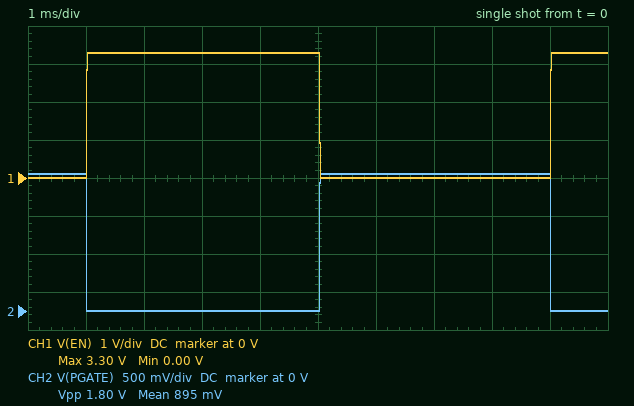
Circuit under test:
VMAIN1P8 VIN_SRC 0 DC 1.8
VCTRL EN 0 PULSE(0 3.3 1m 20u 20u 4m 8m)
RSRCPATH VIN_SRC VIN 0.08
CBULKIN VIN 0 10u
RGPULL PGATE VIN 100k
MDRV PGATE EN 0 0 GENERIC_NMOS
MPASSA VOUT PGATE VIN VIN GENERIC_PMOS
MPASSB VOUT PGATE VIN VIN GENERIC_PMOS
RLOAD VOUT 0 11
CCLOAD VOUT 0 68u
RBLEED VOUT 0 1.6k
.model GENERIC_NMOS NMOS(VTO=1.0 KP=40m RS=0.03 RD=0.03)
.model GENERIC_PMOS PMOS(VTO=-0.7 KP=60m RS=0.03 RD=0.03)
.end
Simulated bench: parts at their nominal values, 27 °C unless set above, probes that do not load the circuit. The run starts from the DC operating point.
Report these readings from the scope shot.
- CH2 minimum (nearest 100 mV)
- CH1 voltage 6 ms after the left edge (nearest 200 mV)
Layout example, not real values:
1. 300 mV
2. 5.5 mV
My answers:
1. 0 V
2. 0 V
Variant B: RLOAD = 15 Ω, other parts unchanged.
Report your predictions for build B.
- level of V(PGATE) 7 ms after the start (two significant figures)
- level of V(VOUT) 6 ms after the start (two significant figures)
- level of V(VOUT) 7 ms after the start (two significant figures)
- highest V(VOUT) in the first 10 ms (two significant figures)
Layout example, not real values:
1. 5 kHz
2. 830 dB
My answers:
1. 1.8 V
2. 380 mV
3. 140 mV
4. 990 mV
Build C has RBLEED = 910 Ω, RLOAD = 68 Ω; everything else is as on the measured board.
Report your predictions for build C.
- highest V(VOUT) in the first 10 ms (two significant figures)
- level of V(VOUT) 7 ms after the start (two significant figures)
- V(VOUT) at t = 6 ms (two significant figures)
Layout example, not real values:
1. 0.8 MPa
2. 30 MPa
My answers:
1. 1.6 V
2. 1.0 V
3. 1.3 V
